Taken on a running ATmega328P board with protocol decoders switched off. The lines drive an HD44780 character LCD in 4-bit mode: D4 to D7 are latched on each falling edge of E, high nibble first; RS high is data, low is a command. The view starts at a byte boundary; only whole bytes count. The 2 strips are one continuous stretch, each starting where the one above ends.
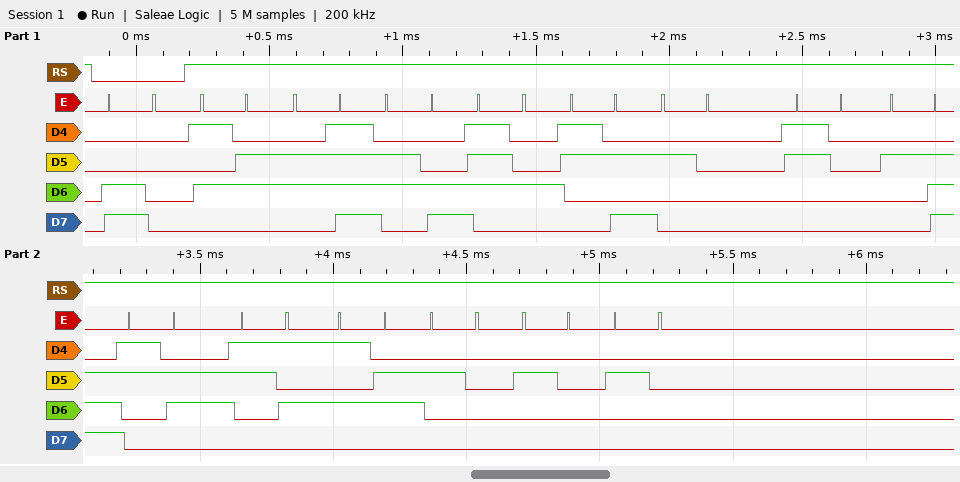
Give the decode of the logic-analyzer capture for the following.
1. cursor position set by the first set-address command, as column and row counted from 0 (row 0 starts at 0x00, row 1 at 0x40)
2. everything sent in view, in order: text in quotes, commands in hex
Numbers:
column 0, row 1
0xC0 "Volt: 0.65V   "
